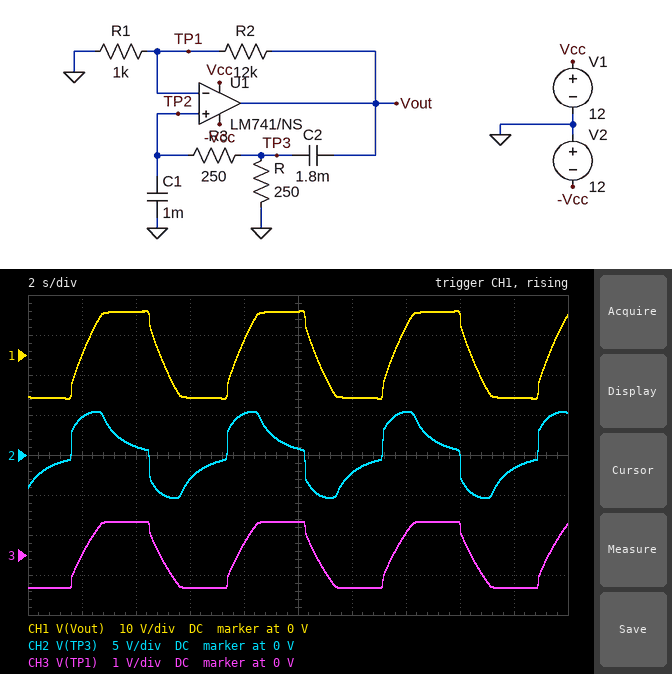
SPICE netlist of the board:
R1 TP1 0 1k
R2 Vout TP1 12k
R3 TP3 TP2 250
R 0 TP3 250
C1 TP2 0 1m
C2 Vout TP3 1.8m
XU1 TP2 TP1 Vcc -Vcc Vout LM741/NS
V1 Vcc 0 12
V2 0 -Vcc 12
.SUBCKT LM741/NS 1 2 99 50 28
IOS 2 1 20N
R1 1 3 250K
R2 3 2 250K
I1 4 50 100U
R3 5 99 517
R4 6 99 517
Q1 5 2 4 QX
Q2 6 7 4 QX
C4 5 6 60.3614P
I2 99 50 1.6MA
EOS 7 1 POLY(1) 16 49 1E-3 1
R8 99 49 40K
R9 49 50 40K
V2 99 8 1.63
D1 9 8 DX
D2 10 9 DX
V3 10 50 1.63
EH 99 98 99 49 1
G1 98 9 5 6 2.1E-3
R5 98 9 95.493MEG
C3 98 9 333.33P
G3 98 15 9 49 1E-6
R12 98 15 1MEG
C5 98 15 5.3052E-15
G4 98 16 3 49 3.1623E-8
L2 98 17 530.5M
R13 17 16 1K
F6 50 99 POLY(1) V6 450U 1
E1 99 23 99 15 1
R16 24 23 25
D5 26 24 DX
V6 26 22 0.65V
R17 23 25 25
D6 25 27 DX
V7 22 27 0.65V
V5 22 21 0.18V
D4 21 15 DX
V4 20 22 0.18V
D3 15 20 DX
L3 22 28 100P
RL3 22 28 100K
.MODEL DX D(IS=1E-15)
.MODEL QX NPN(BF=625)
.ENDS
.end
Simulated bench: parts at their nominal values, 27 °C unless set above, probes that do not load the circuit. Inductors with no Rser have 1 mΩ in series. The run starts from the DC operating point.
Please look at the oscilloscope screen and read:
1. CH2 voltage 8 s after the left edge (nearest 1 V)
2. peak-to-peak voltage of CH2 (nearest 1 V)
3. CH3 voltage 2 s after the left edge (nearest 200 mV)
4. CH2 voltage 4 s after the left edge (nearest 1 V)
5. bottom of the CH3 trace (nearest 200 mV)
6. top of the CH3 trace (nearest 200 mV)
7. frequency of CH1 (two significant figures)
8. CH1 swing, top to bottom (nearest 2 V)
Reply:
5 V
11 V
0 V
1 V
-800 mV
800 mV
170 mHz
22 V
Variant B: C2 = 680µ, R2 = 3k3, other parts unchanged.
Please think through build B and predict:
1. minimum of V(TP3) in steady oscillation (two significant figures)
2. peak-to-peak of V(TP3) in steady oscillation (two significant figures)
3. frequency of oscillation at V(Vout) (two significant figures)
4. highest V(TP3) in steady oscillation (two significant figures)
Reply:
-3.8 V
7.6 V
680 mHz
3.8 V
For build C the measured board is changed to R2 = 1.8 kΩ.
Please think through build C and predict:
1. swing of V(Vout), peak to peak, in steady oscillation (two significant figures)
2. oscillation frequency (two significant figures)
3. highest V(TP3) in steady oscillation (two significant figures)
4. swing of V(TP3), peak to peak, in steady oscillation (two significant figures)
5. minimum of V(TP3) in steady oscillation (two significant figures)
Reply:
21 V
330 mHz
4.7 V
9.4 V
-4.7 V
